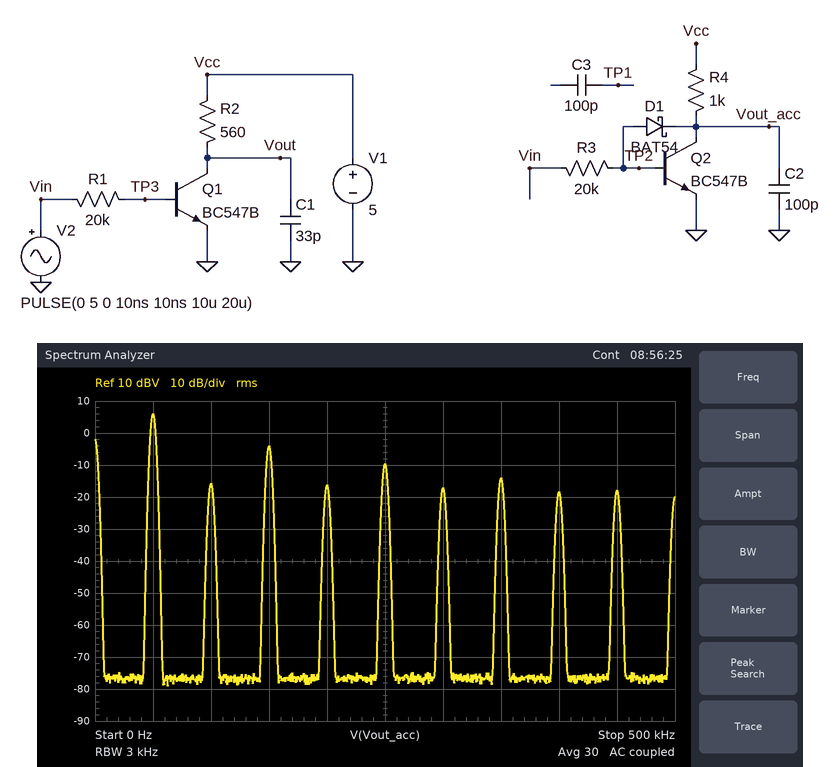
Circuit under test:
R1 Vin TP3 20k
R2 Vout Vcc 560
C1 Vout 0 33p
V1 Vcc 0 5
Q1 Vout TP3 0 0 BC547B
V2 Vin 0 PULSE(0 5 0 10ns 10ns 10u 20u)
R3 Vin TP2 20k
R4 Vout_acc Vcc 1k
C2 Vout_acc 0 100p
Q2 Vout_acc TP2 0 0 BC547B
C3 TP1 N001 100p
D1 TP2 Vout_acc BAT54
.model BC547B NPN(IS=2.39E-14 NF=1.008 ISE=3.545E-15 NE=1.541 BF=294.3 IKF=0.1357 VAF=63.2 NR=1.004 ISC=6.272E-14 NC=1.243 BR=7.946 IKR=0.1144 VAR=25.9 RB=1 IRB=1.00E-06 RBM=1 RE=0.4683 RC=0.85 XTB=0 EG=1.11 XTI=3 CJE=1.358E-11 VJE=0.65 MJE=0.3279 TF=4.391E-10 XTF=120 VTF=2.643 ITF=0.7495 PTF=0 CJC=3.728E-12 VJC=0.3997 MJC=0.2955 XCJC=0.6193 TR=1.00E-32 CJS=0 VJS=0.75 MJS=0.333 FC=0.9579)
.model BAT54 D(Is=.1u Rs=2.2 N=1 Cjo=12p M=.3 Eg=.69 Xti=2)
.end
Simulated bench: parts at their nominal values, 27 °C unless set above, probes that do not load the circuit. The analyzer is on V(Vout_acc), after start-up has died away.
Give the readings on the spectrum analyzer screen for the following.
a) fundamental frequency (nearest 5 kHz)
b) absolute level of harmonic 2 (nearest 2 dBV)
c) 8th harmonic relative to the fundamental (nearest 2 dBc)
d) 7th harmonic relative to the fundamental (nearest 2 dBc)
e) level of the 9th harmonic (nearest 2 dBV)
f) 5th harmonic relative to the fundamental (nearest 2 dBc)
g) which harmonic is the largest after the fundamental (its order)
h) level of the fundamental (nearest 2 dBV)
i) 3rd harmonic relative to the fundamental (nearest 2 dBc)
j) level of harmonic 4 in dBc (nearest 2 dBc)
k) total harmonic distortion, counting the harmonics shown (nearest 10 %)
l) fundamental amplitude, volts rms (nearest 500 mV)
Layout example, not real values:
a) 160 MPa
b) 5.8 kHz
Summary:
a) 50 kHz
b) -16 dBV
c) -24 dBc
d) -20 dBc
e) -18 dBV
f) -16 dBc
g) 3
h) 6 dBV
i) -10 dBc
j) -22 dBc
k) 40 %
l) 2.0 V
